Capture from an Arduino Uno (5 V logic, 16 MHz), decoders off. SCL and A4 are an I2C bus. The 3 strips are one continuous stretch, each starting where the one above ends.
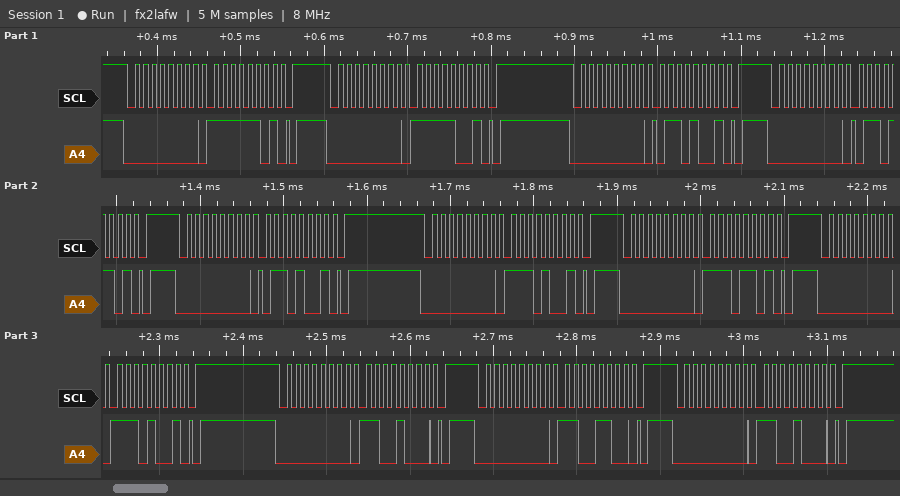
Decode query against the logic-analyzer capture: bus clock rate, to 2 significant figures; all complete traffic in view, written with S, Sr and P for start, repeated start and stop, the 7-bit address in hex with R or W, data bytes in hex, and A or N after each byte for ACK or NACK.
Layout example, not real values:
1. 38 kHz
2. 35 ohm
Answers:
1. 100 kHz
2. S 00W A FD A P S 00W A F9 A P S 00W A 69 A P S 00W A 6D A P S 00W A 69 A P S 00W A E9 A P S 00W A ED A P S 00W A E9 A P S 00W A C8 A P S 00W A CC A P S 00W A C8 A P
